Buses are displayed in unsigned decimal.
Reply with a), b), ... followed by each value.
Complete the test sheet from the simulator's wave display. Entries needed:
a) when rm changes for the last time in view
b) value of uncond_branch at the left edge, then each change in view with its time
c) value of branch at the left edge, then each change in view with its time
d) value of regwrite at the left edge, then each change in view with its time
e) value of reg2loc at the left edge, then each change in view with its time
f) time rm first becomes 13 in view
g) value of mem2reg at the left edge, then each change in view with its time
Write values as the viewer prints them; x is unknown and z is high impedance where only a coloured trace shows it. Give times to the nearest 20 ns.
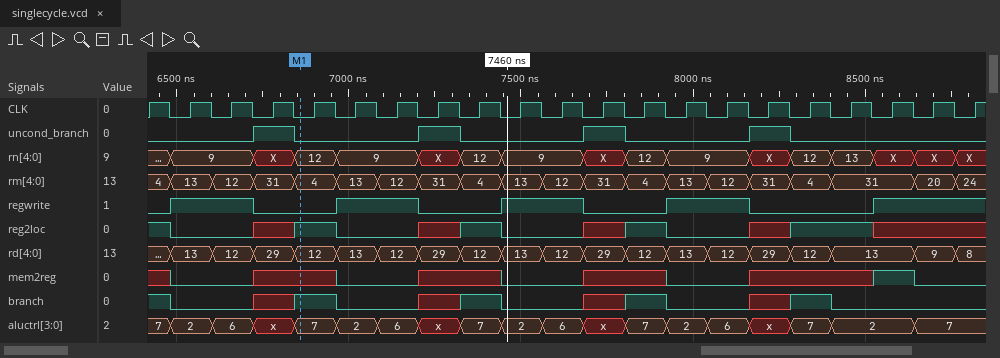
a) 8760 ns
b) 0, 1 at 6720 ns, 0 at 6840 ns, 1 at 7200 ns, 0 at 7320 ns, 1 at 7680 ns, 0 at 7800 ns, 1 at 8160 ns, 0 at 8280 ns
c) 1, 0 at 6480 ns, x at 6720 ns, 1 at 6840 ns, 0 at 6960 ns, x at 7200 ns, 1 at 7320 ns, 0 at 7440 ns, x at 7680 ns, 1 at 7800 ns, 0 at 7920 ns, x at 8160 ns, 1 at 8280 ns, 0 at 8400 ns
d) 0, 1 at 6480 ns, 0 at 6720 ns, 1 at 6960 ns, 0 at 7200 ns, 1 at 7440 ns, 0 at 7680 ns, 1 at 7920 ns, 0 at 8160 ns, 1 at 8520 ns
e) 1, 0 at 6480 ns, x at 6720 ns, 1 at 6840 ns, 0 at 6960 ns, x at 7200 ns, 1 at 7320 ns, 0 at 7440 ns, x at 7680 ns, 1 at 7800 ns, 0 at 7920 ns, x at 8160 ns, 1 at 8280 ns, x at 8520 ns
f) 6480 ns
g) x, 0 at 6480 ns, x at 6720 ns, 0 at 6960 ns, x at 7200 ns, 0 at 7440 ns, x at 7680 ns, 0 at 7920 ns, x at 8160 ns, 1 at 8520 ns, 0 at 8640 ns
